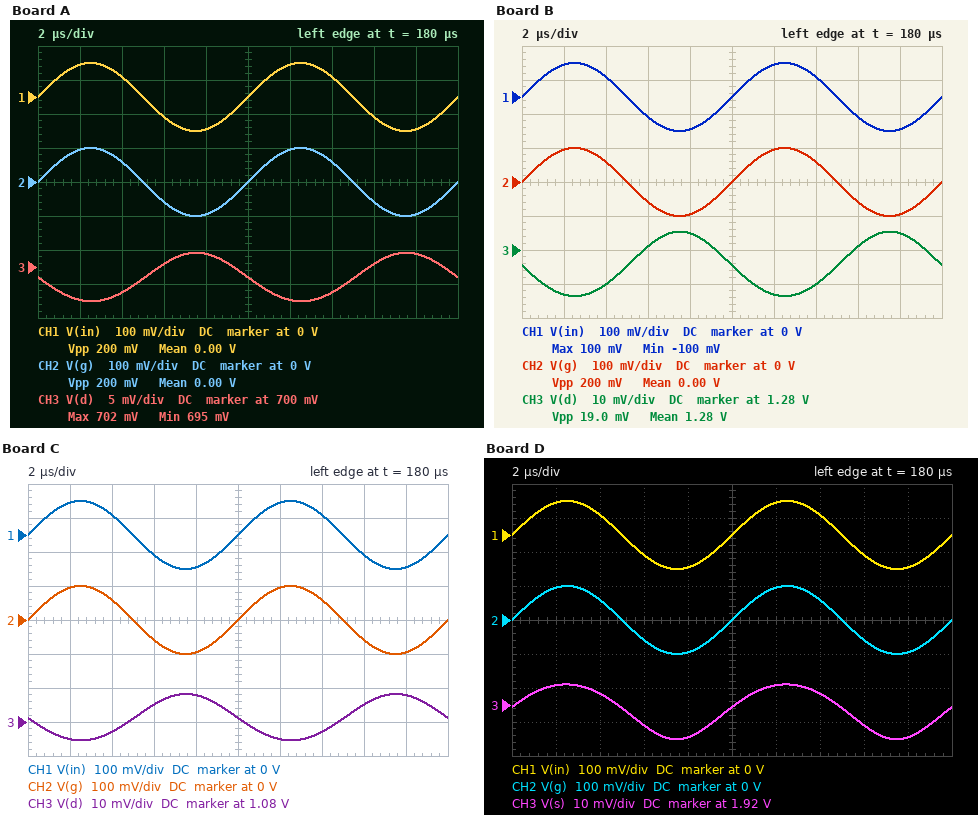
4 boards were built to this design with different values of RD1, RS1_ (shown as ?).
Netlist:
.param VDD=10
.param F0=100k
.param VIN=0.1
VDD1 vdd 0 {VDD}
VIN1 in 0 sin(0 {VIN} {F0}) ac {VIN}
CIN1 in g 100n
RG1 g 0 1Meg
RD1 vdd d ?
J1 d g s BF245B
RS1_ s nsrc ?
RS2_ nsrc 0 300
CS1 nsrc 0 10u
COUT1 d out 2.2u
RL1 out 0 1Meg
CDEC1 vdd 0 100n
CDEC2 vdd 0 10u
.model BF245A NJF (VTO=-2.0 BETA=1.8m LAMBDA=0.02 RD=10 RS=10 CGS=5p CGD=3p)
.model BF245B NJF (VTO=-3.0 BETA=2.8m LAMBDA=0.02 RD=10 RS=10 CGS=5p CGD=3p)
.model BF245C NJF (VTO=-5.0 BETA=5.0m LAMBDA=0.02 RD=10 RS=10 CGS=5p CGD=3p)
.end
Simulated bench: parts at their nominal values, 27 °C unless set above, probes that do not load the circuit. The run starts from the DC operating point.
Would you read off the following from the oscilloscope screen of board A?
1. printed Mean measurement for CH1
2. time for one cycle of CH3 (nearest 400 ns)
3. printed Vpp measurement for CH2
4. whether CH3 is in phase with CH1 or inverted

0.00 V
10.0 µs
200 mV
inverted
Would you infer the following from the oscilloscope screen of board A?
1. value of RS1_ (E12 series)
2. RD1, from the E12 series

220 Ω
8.2 kΩ
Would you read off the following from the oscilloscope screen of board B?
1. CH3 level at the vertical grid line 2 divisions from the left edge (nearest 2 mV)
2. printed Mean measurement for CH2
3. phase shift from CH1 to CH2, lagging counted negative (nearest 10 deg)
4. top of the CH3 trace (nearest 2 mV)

1.270 V
0.00 V
0 deg
1.286 V
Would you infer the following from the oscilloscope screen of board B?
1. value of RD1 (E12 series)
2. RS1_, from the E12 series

4.7 kΩ
270 Ω
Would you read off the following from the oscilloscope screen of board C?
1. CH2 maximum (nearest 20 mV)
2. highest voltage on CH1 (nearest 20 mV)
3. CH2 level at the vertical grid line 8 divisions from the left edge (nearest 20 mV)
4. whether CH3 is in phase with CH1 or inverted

100 mV
100 mV
-60 mV
inverted
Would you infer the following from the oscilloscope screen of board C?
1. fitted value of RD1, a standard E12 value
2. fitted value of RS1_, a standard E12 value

5.6 kΩ
270 Ω
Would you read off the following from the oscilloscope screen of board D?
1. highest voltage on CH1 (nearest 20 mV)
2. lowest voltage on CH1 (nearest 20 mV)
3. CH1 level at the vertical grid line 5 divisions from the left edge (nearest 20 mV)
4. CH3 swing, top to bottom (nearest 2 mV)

100 mV
-100 mV
0 V
16 mV
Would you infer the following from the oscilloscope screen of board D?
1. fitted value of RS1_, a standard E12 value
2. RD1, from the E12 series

680 Ω
3.9 kΩ
